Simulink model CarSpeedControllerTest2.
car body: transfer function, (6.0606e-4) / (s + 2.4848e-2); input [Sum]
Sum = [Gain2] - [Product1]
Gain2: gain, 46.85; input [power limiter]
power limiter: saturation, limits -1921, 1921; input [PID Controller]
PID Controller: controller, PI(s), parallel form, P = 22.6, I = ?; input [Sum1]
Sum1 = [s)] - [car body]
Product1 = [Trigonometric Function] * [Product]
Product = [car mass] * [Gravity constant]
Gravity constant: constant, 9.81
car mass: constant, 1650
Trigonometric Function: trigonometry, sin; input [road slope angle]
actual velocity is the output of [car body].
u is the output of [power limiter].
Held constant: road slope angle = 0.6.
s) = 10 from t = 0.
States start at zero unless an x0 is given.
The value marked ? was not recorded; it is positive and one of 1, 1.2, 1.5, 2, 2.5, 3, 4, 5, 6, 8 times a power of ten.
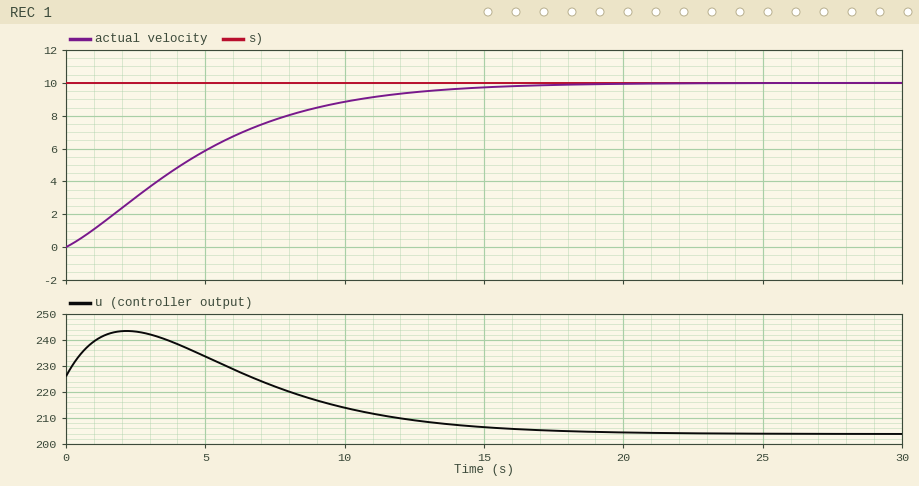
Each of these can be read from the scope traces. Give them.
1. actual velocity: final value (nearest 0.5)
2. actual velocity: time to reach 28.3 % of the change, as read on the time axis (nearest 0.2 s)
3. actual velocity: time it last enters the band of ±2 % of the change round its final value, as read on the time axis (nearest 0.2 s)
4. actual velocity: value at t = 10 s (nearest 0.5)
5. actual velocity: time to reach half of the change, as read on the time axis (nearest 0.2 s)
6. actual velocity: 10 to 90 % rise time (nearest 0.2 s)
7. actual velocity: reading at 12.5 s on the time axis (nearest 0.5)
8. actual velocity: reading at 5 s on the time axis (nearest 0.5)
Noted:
10.0
2.4 s
16.0 s
9.0
4.2 s
9.6 s
9.5
6.0
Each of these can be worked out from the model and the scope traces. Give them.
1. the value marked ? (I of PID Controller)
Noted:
4
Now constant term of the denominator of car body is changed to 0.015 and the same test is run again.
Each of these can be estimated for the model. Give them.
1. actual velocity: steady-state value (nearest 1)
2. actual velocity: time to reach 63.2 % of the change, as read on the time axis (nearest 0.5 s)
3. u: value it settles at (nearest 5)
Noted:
10
5.5 s
200
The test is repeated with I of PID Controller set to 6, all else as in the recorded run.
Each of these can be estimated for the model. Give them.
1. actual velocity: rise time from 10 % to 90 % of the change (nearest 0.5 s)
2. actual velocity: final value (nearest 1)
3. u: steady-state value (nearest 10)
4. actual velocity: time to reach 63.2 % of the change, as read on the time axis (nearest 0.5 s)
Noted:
6.0 s
10
200
4.0 s
